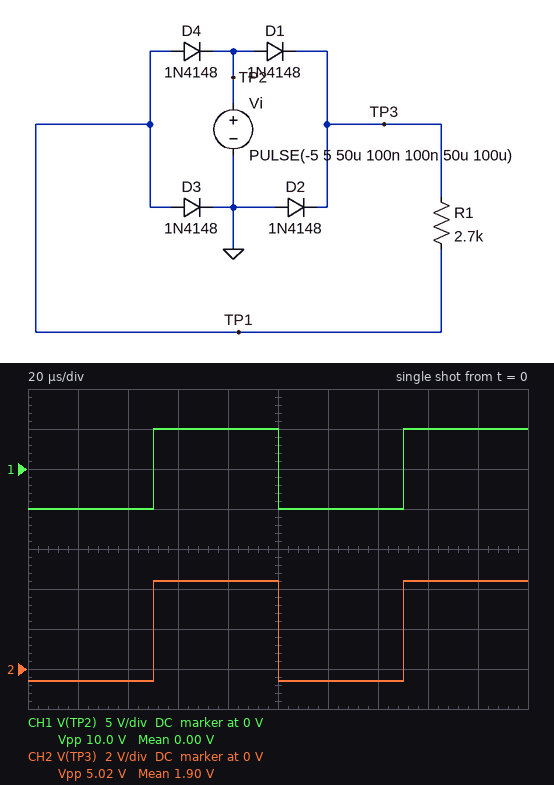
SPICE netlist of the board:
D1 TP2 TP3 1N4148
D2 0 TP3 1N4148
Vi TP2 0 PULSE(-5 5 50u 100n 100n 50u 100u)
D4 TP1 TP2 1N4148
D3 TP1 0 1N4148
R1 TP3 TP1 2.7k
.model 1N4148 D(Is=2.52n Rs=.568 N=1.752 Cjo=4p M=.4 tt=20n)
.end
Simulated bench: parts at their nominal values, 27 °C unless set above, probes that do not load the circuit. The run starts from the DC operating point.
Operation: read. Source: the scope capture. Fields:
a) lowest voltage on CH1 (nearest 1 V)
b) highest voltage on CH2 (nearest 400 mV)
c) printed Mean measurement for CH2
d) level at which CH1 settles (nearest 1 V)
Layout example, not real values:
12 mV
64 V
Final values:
-5 V
4.4 V
1.90 V
5 V
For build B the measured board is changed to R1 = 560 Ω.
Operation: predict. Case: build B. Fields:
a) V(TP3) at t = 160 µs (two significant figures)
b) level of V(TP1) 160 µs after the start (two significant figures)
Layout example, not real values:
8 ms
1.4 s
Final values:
4.3 V
670 mV
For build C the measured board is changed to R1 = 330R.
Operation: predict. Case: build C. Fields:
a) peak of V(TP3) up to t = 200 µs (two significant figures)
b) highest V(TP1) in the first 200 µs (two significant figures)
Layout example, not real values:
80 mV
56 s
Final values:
4.3 V
700 mV
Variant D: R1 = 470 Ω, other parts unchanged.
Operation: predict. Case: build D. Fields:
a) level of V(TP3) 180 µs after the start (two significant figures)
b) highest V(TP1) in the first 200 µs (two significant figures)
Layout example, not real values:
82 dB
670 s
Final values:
4.3 V
680 mV
